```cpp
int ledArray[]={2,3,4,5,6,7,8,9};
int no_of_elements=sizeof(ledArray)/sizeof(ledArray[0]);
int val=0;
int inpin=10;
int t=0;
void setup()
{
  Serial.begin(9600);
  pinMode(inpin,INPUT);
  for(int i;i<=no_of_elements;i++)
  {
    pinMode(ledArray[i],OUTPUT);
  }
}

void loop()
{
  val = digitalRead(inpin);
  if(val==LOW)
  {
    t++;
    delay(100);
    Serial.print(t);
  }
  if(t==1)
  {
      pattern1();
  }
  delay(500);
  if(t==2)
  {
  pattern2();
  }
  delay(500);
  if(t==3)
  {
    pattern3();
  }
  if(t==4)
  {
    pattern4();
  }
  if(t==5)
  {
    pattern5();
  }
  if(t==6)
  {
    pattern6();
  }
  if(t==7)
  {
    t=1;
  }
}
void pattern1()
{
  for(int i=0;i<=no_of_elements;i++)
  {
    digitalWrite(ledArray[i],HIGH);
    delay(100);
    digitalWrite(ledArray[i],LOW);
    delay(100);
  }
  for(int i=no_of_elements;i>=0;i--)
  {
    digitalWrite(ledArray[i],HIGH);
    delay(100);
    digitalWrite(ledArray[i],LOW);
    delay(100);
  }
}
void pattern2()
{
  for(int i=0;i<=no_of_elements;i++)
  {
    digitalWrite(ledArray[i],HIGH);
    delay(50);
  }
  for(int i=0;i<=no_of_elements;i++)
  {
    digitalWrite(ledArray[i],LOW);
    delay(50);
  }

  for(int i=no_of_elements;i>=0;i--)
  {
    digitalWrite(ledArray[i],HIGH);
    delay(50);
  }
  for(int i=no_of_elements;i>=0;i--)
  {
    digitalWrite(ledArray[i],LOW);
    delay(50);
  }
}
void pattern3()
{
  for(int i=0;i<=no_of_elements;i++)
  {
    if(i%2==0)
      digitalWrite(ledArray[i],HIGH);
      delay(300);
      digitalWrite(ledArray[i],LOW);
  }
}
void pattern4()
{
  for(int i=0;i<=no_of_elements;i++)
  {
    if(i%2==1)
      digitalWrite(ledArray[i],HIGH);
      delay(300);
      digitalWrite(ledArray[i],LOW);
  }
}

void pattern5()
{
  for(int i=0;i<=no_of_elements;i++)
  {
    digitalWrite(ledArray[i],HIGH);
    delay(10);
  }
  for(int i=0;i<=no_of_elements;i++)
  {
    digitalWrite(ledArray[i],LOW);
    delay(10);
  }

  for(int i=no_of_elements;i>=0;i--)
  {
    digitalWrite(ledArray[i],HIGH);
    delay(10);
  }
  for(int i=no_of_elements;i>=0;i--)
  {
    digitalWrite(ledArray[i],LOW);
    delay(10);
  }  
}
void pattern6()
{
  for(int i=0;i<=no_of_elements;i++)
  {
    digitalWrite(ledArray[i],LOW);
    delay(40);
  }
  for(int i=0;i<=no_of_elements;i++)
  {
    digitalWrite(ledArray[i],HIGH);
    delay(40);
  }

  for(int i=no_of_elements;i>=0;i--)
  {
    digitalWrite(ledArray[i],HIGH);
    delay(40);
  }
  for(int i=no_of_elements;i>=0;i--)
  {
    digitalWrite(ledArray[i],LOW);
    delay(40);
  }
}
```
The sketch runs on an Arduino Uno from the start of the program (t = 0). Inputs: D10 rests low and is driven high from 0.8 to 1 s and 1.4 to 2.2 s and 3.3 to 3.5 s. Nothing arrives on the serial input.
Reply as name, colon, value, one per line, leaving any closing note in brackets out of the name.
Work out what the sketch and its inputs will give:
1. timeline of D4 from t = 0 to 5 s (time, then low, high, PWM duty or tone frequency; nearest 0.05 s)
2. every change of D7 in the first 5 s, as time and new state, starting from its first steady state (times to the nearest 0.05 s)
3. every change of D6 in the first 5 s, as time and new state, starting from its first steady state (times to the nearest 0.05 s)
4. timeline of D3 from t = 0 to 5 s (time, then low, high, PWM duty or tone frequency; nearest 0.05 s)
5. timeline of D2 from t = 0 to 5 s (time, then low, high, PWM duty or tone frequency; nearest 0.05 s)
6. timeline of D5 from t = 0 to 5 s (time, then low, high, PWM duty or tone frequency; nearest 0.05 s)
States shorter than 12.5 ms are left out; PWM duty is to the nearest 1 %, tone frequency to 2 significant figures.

timeline of D4 from t = 0 to 5 s: 0 s low; 0.5 s high; 0.6 s low; 3.1 s high; 3.2 s low
every change of D7 in the first 5 s, as time and new state, starting from its first steady state: 0 s low; 1.1 s high; 1.2 s low; 2.5 s high; 2.6 s low
every change of D6 in the first 5 s, as time and new state, starting from its first steady state: 0 s low; 0.9 s high; 1 s low; 2.7 s high; 2.8 s low
timeline of D3 from t = 0 to 5 s: 0 s low; 0.3 s high; 0.4 s low; 3.3 s high; 3.4 s low
timeline of D2 from t = 0 to 5 s: 0 s low; 0.1 s high; 0.2 s low; 3.5 s high; 3.6 s low
timeline of D5 from t = 0 to 5 s: 0 s low; 0.7 s high; 0.8 s low; 2.9 s high; 3 s low
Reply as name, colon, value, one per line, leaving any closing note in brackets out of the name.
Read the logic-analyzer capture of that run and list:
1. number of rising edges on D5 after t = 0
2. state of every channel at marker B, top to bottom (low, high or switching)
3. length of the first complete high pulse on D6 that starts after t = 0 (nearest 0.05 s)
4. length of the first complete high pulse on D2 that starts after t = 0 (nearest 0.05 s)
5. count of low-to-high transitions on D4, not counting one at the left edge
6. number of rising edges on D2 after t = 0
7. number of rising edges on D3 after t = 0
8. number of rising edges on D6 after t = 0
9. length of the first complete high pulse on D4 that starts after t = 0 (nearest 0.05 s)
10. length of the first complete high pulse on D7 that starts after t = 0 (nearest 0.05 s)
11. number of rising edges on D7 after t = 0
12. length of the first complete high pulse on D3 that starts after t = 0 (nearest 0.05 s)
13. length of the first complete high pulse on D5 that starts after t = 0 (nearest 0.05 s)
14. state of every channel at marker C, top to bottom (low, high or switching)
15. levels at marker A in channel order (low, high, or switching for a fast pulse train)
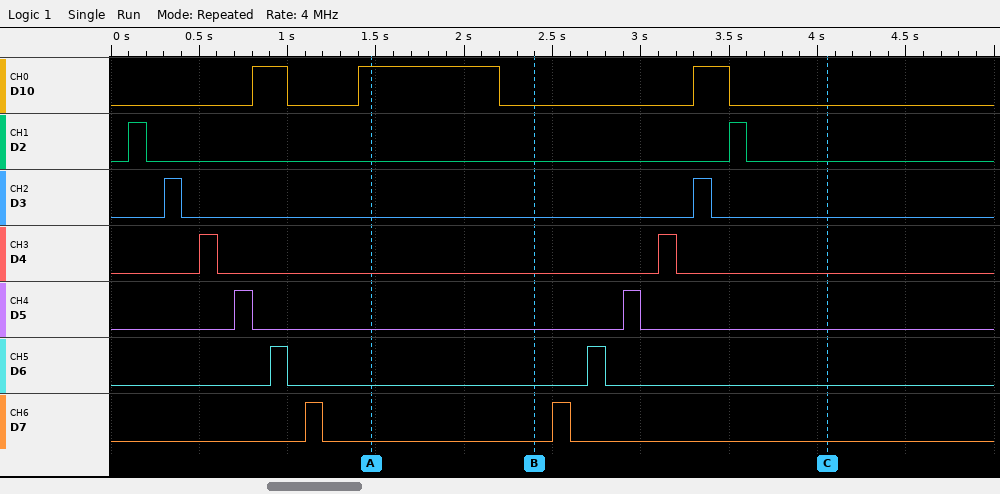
number of rising edges on D5 after t = 0: 2
state of every channel at marker B, top to bottom: D10 low, D2 low, D3 low, D4 low, D5 low, D6 low, D7 low
length of the first complete high pulse on D6 that starts after t = 0: 0.10 s
length of the first complete high pulse on D2 that starts after t = 0: 0.10 s
count of low-to-high transitions on D4, not counting one at the left edge: 2
number of rising edges on D2 after t = 0: 2
number of rising edges on D3 after t = 0: 2
number of rising edges on D6 after t = 0: 2
length of the first complete high pulse on D4 that starts after t = 0: 0.10 s
length of the first complete high pulse on D7 that starts after t = 0: 0.10 s
number of rising edges on D7 after t = 0: 2
length of the first complete high pulse on D3 that starts after t = 0: 0.10 s
length of the first complete high pulse on D5 that starts after t = 0: 0.10 s
state of every channel at marker C, top to bottom: D10 low, D2 low, D3 low, D4 low, D5 low, D6 low, D7 low
levels at marker A in channel order: D10 high, D2 low, D3 low, D4 low, D5 low, D6 low, D7 low
